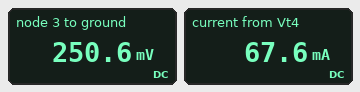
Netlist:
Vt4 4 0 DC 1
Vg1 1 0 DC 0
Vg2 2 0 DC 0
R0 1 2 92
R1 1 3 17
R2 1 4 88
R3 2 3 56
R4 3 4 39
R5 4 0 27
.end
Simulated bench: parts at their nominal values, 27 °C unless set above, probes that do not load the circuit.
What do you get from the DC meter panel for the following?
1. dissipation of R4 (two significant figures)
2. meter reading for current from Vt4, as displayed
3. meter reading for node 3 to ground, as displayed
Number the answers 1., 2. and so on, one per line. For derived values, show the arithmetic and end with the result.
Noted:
1. (1 V - 250.6 mV)^2 / 39 Ω = 14 mW
2. 67.6 mA
3. 250.6 mV
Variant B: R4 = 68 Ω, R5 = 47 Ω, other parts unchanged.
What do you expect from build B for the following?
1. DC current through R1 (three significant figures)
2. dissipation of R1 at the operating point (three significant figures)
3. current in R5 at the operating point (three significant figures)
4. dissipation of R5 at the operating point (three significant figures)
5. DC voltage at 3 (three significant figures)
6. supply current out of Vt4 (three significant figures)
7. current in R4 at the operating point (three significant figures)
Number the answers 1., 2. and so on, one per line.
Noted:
1. 9.47 mA
2. 1.52 mW
3. 21.3 mA
4. 21.3 mW
5. 161 mV
6. 45.0 mA
7. 12.3 mA
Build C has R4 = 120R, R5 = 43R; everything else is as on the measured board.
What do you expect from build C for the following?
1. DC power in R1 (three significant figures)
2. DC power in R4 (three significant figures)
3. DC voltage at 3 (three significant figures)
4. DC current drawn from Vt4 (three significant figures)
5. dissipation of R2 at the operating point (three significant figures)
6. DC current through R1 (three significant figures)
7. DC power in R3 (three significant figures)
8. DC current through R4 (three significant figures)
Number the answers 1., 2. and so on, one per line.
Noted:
1. 565 µW
2. 6.78 mW
3. 98.0 mV
4. 42.1 mA
5. 11.4 mW
6. 5.77 mA
7. 172 µW
8. 7.52 mA
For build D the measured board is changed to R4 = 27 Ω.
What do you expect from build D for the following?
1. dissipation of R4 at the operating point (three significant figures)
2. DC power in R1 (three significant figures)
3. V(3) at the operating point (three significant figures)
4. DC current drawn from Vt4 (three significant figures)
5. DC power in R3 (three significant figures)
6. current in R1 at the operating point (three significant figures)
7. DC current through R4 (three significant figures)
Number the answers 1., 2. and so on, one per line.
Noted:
1. 16.8 mW
2. 6.24 mW
3. 326 mV
4. 73.4 mA
5. 1.89 mW
6. 19.2 mA
7. 25.0 mA
